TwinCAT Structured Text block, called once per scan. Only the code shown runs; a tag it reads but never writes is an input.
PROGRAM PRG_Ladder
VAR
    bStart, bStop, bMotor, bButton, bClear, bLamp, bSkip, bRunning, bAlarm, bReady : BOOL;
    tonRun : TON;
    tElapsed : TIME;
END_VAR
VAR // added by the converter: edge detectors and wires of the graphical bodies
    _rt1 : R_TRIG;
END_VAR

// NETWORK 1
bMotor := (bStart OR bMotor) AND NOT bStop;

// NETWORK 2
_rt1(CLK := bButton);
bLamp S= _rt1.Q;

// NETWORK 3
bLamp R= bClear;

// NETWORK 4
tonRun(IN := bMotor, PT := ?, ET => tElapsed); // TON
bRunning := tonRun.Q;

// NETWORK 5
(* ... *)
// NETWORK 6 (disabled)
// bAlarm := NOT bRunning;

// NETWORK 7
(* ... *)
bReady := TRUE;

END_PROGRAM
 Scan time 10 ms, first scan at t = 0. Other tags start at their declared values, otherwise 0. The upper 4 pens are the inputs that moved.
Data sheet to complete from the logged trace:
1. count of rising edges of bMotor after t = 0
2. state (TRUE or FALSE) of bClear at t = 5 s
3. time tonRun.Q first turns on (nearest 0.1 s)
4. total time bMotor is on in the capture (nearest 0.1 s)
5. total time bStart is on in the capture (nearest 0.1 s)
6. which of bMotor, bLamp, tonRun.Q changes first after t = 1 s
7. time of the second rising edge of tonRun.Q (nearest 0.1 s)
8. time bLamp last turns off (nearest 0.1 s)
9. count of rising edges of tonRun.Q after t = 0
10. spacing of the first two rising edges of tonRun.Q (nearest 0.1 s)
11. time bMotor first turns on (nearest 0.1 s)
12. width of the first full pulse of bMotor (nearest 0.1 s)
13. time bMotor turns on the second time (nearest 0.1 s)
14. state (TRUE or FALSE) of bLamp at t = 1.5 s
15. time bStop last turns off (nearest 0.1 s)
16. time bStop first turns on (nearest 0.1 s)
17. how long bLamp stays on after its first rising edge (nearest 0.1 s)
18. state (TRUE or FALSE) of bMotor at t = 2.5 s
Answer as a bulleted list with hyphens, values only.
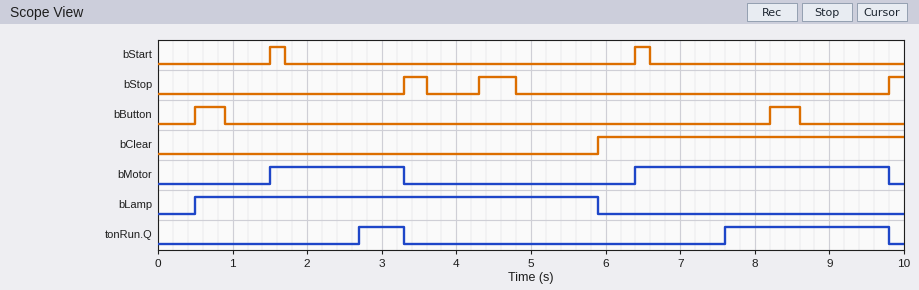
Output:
- 2
- FALSE
- 2.7 s
- 5.2 s
- 0.4 s
- bMotor
- 7.6 s
- 5.9 s
- 2
- 4.9 s
- 1.5 s
- 1.8 s
- 6.4 s
- TRUE
- 4.8 s
- 3.3 s
- 5.4 s
- TRUE
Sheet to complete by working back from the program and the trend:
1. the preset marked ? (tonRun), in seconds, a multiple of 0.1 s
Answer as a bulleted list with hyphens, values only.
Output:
- 1.2 s
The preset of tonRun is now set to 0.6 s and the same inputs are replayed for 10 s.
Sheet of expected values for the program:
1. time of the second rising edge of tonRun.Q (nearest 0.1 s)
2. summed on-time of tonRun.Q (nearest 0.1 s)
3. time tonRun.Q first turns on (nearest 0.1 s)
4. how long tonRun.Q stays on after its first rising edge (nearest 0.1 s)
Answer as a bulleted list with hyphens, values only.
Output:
- 7.0 s
- 4.0 s
- 2.1 s
- 1.2 s
